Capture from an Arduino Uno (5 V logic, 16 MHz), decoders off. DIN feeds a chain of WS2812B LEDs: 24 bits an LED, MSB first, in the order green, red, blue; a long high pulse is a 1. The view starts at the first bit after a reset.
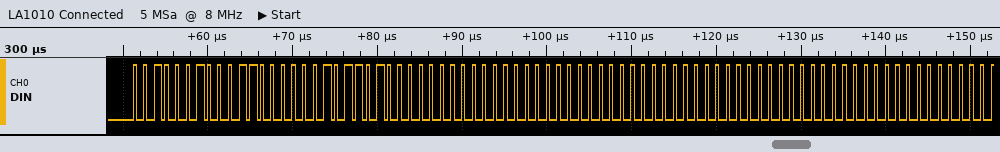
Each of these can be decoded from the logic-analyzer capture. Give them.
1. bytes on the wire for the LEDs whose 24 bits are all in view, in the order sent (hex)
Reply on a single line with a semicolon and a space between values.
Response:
22 30 2D 00 00 00 00 00 00
